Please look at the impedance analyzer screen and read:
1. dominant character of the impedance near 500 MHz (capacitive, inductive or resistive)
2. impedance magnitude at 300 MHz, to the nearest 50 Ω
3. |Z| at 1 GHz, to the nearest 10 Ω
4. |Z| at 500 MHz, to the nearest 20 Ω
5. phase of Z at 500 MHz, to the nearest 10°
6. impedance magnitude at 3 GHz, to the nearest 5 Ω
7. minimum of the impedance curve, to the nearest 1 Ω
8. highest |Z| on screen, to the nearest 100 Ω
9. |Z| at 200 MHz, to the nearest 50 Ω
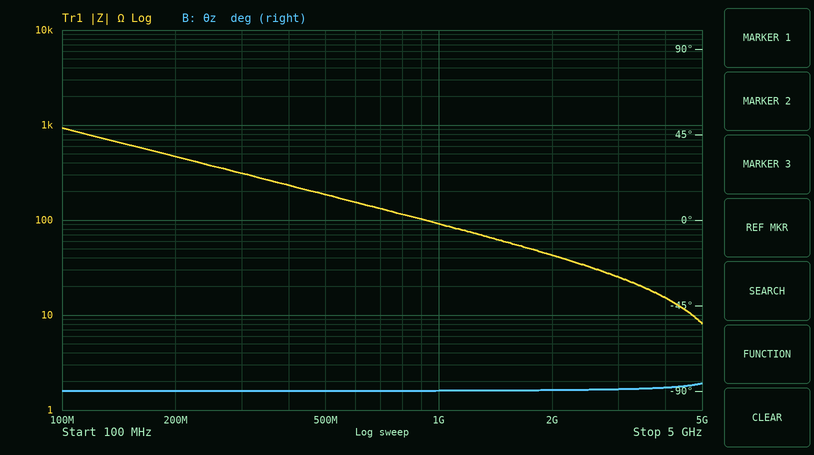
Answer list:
capacitive
300 Ω
90 Ω
180 Ω
-90°
25 Ω
8 Ω
900 Ω
450 Ω
